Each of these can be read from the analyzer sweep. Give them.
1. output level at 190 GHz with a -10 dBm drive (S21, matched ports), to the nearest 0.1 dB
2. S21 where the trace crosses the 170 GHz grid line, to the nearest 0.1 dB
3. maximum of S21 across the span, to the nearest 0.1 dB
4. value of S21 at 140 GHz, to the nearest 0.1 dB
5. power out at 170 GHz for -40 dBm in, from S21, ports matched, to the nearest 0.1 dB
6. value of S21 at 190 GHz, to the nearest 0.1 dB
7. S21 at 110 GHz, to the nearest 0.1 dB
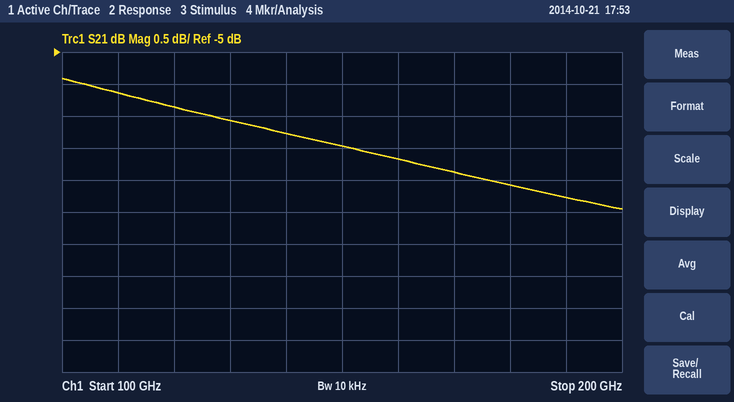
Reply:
-17.3 dBm
-6.9 dB
-5.4 dB
-6.3 dB
-46.9 dBm
-7.3 dB
-5.6 dB
